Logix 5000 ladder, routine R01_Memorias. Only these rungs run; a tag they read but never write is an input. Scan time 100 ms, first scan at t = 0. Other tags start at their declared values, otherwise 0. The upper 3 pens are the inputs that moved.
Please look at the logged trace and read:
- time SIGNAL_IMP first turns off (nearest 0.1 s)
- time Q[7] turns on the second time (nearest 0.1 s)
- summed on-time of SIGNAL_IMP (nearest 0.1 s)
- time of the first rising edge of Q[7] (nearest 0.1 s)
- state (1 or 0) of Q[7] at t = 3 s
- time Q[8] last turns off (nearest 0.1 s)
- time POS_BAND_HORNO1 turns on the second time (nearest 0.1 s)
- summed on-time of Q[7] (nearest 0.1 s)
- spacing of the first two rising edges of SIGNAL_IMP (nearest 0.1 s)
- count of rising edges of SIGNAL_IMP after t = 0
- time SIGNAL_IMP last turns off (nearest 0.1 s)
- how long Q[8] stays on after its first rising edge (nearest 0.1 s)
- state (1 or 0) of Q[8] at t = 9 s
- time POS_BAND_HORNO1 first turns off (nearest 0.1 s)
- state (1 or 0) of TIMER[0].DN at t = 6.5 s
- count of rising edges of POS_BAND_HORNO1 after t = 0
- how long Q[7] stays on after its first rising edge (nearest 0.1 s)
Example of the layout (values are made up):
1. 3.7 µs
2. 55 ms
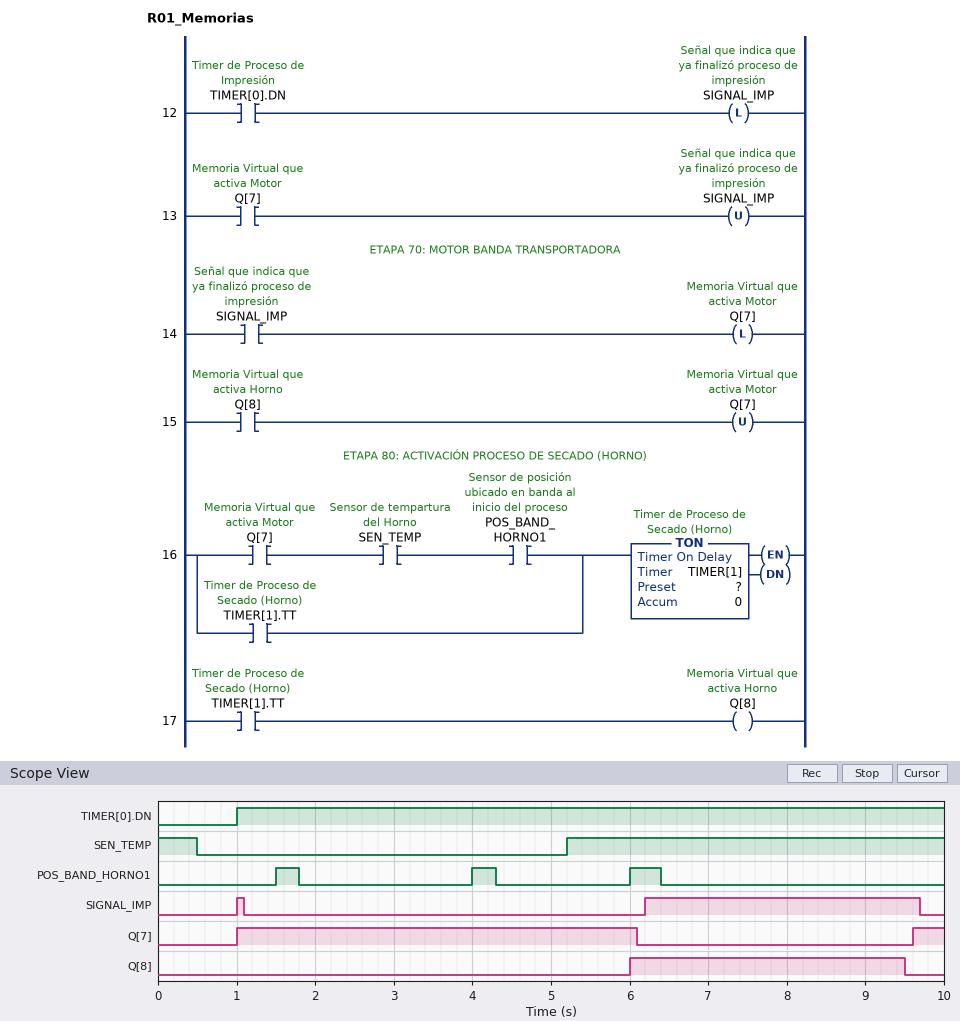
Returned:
1. 1.1 s
2. 9.6 s
3. 3.6 s
4. 1.0 s
5. 1
6. 9.5 s
7. 4.0 s
8. 5.5 s
9. 5.2 s
10. 2
11. 9.7 s
12. 3.5 s
13. 1
14. 1.8 s
15. 1
16. 3
17. 5.1 s
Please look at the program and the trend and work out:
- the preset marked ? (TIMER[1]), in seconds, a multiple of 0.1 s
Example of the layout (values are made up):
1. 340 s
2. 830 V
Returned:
1. 3.5 s
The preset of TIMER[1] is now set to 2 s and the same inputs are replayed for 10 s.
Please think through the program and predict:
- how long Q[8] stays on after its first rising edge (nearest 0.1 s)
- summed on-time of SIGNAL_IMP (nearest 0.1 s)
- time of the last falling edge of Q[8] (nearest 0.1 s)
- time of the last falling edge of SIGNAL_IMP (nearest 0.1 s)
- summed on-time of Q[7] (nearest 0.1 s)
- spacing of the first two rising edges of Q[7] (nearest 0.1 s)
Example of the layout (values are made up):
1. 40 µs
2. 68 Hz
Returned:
1. 2.0 s
2. 2.1 s
3. 8.0 s
4. 8.2 s
5. 7.0 s
6. 7.1 s
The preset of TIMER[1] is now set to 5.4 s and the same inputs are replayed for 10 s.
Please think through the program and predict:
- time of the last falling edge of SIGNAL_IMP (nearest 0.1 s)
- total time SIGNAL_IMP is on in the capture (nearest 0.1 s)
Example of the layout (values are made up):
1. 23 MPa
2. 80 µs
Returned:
1. 1.1 s
2. 3.9 s
